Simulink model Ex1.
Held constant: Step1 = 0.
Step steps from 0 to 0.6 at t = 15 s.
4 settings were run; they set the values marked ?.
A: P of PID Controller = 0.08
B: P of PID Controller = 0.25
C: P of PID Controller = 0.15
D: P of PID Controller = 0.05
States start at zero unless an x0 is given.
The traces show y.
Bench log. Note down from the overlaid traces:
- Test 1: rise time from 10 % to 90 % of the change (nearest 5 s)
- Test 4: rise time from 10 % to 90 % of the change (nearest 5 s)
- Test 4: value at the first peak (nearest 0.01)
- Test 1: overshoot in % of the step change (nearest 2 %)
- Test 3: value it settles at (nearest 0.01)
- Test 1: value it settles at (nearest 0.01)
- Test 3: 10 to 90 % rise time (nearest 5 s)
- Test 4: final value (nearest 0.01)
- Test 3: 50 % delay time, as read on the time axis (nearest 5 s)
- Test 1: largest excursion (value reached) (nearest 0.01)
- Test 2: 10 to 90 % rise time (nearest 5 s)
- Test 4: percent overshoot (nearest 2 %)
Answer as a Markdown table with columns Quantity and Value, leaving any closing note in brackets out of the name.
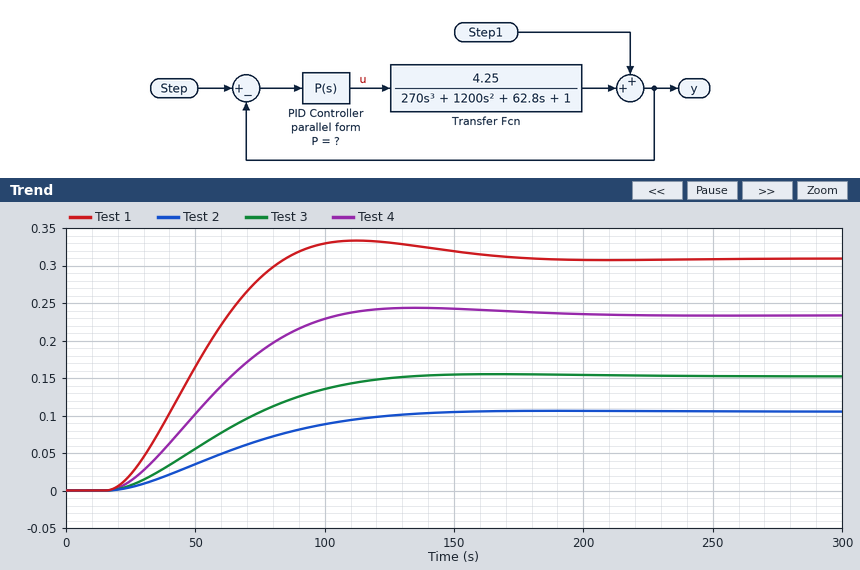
| Quantity | Value |
|---|---|
| Test 1: rise time from 10 % to 90 % of the change | 45 s |
| Test 4: rise time from 10 % to 90 % of the change | 60 s |
| Test 4: value at the first peak | 0.24 |
| Test 1: overshoot in % of the step change | 8 % |
| Test 3: value it settles at | 0.15 |
| Test 1: value it settles at | 0.31 |
| Test 3: 10 to 90 % rise time | 70 s |
| Test 4: final value | 0.23 |
| Test 3: 50 % delay time, as read on the time axis | 60 s |
| Test 1: largest excursion (value reached) | 0.33 |
| Test 2: 10 to 90 % rise time | 80 s |
| Test 4: percent overshoot | 4 % |
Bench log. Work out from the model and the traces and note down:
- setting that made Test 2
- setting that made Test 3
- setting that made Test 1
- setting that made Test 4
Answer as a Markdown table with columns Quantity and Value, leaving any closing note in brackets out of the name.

| Quantity | Value |
|---|---|
| setting that made Test 2 | D |
| setting that made Test 3 | A |
| setting that made Test 1 | B |
| setting that made Test 4 | C |
